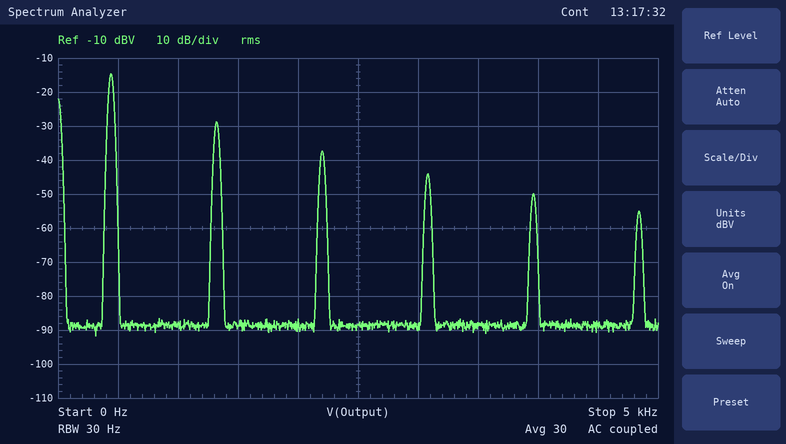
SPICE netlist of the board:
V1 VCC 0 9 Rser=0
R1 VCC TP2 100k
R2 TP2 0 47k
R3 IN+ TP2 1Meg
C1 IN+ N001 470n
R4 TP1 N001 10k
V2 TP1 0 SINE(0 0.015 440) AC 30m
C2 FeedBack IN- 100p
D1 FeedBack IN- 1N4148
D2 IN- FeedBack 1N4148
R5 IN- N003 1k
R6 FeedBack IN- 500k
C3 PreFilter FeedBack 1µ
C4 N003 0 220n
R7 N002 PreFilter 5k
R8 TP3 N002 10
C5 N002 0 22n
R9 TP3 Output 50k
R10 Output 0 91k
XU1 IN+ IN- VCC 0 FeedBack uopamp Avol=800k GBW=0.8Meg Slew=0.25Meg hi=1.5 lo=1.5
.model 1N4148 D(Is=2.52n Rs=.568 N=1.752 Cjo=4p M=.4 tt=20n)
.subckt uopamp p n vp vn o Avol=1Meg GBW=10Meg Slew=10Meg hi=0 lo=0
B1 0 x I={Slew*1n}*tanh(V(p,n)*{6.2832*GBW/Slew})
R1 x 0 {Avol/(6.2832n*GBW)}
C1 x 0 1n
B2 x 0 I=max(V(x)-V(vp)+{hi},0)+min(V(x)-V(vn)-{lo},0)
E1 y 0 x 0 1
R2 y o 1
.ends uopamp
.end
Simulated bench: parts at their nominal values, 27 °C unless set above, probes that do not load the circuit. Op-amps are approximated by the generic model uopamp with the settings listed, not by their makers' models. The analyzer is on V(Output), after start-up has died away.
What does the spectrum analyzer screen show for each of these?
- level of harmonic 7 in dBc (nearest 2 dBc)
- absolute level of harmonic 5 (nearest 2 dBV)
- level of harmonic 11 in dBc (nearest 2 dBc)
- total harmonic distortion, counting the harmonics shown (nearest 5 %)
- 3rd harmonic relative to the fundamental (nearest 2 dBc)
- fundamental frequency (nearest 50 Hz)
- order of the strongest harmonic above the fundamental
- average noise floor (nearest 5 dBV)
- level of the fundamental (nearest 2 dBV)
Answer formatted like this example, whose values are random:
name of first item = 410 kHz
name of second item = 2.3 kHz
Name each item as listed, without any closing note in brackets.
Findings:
level of harmonic 7 in dBc = -30 dBc
absolute level of harmonic 5 = -38 dBV
level of harmonic 11 in dBc = -40 dBc
total harmonic distortion, counting the harmonics shown = 20 %
3rd harmonic relative to the fundamental = -14 dBc
fundamental frequency = 450 Hz
order of the strongest harmonic above the fundamental = 3
average noise floor = -90 dBV
level of the fundamental = -14 dBV
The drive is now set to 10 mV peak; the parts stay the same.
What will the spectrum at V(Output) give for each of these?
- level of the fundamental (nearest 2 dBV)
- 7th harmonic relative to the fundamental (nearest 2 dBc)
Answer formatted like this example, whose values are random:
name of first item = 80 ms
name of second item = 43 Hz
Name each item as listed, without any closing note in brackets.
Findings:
level of the fundamental = -16 dBV
7th harmonic relative to the fundamental = -30 dBc
